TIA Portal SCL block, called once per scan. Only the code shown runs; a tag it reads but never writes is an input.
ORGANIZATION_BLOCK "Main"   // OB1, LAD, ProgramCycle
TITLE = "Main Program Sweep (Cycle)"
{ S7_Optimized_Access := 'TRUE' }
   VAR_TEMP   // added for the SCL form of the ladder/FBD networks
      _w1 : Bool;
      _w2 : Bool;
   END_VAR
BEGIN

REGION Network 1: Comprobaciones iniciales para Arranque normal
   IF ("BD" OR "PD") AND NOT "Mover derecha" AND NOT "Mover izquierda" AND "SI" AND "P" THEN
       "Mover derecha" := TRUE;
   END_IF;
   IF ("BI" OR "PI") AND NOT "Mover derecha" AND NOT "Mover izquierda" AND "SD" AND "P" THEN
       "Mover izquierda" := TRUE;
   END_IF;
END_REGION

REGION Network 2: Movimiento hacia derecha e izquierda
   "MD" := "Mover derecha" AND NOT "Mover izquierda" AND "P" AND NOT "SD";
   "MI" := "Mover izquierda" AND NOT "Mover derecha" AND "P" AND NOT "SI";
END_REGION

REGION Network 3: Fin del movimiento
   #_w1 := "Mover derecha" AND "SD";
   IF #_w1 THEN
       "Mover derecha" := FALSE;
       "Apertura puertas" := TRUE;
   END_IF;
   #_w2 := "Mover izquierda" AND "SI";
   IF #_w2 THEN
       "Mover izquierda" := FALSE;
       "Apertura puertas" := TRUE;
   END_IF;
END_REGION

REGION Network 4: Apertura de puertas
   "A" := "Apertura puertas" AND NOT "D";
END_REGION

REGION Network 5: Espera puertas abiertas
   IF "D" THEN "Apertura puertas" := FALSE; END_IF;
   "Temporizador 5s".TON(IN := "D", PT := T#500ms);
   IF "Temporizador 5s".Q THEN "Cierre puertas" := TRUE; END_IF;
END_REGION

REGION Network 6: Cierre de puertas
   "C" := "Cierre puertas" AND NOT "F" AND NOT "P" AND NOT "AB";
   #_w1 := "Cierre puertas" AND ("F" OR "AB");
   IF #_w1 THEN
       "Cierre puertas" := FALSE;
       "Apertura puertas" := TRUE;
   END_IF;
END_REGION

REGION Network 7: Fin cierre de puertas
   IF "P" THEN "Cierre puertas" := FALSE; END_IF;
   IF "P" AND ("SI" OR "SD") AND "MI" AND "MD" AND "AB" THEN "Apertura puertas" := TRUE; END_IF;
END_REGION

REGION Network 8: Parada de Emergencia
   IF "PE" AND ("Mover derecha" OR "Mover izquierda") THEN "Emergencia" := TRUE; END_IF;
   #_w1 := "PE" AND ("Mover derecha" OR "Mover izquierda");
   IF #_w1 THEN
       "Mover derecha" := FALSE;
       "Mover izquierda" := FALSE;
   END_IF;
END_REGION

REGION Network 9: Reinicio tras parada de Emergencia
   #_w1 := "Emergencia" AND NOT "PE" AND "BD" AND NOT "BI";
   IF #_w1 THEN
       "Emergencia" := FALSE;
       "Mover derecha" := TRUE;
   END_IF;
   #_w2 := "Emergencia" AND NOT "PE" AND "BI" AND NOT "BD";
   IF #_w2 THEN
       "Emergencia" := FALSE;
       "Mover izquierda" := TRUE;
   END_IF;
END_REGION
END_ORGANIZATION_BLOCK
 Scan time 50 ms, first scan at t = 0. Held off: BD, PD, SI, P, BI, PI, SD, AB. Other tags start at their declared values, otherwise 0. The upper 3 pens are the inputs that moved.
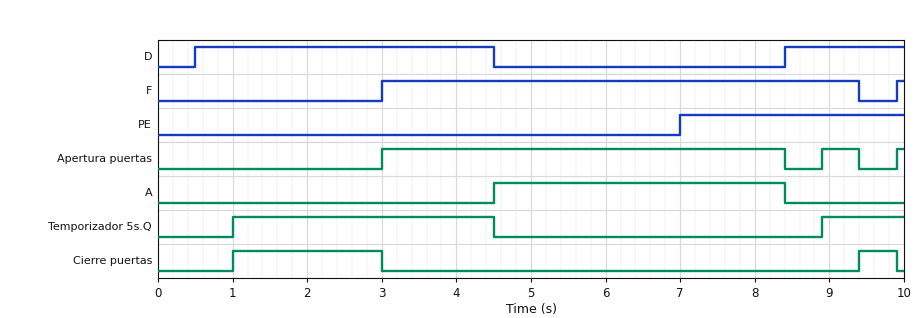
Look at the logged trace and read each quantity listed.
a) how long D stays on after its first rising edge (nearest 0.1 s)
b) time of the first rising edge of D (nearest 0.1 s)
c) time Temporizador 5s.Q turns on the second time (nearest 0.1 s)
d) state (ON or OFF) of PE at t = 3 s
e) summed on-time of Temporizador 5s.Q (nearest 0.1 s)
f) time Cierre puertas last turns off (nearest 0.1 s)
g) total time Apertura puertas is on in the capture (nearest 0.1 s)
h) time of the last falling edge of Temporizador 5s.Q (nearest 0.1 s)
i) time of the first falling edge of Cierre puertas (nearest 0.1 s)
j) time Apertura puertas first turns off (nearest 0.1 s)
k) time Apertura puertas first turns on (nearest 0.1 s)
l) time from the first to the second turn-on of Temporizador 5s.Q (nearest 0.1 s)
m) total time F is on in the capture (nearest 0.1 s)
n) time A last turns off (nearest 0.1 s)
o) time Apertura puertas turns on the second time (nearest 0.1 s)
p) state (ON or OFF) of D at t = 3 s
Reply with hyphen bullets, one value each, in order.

- 4.0 s
- 0.5 s
- 8.9 s
- OFF
- 4.6 s
- 9.9 s
- 6.0 s
- 4.5 s
- 3.0 s
- 8.4 s
- 3.0 s
- 7.9 s
- 6.5 s
- 8.4 s
- 8.9 s
- ON
